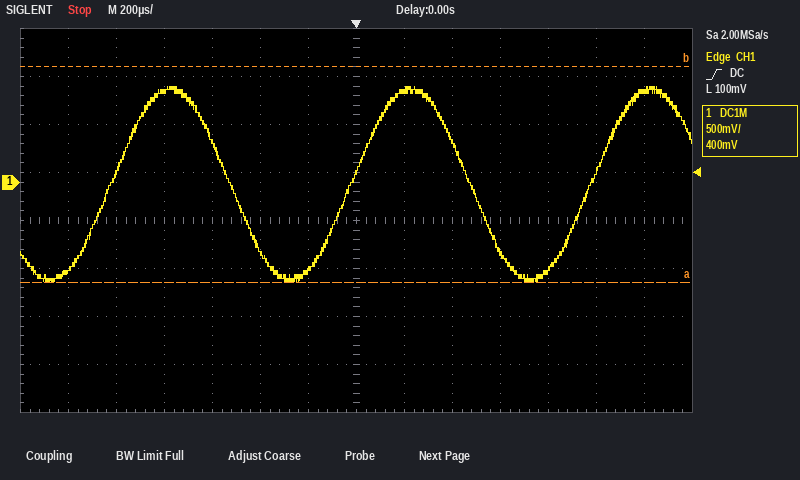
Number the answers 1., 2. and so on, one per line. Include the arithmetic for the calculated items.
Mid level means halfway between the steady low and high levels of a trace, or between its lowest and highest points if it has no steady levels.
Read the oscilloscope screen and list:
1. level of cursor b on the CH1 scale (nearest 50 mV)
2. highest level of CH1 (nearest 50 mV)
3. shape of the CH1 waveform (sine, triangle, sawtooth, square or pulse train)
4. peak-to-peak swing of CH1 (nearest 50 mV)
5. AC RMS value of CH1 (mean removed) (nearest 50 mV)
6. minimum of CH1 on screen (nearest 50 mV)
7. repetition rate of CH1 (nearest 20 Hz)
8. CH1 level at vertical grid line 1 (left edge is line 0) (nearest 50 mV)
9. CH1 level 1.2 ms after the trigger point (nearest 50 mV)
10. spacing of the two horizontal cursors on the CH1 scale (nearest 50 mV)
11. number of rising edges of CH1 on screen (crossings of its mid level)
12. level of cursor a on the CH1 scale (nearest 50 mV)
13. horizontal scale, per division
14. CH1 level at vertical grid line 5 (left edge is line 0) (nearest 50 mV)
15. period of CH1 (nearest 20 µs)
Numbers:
1. 1.20 V
2. 1.00 V
3. sine
4. 1.00 V − (-1.05 V) = 2.05 V
5. 2.05 V / (2√2) ≈ 725 mV, so 700 mV to the nearest 50 mV
6. -1.05 V
7. 1 / 1.00 ms ≈ 1.00 kHz
8. -900 mV
9. 950 mV
10. 2.25 V
11. 3
12. -1.05 V
13. 200 µs
14. -700 mV
15. 1.00 ms
